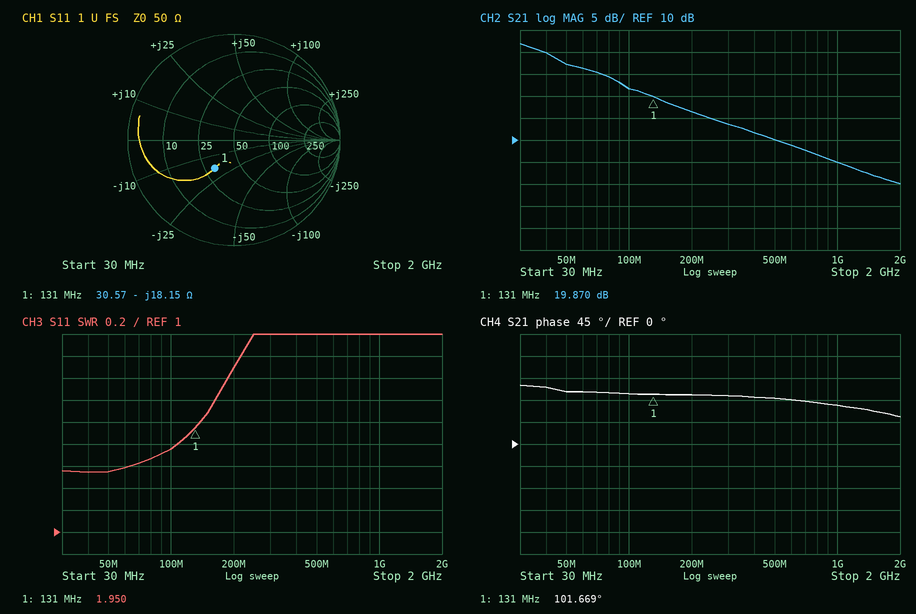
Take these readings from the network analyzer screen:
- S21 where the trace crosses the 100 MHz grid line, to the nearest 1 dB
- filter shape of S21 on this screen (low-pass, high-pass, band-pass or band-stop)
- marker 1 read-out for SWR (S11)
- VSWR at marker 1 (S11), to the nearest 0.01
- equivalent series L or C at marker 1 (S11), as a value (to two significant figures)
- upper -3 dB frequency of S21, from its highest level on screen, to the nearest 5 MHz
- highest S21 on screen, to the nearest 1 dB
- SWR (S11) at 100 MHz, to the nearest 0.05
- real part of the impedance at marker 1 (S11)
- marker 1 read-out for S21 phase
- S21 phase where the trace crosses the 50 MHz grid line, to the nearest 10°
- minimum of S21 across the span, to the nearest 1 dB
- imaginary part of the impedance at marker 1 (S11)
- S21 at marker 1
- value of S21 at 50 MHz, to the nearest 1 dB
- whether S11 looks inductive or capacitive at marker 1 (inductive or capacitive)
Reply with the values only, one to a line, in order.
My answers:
22 dB
low-pass
1.950
1.95
67 pF
45 MHz
32 dB
1.75
30.57 Ω
101.669°
110°
0 dB
-18.15 Ω
19.870 dB
27 dB
capacitive
